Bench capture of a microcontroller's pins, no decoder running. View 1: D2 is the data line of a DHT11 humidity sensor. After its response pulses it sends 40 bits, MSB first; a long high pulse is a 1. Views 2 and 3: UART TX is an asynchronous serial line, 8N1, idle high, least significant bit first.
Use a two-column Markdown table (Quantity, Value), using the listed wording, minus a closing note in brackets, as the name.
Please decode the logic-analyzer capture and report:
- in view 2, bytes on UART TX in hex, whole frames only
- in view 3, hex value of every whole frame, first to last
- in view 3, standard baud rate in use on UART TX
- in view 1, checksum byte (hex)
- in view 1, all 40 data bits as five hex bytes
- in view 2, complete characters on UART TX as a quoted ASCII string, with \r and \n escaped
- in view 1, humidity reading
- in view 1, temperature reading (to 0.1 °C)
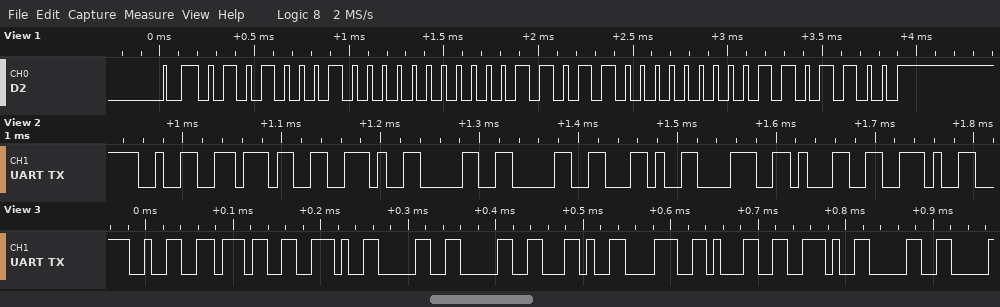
| Quantity | Value |
|---|---|
| in view 2, bytes on UART TX in hex, whole frames only | 32 37 2E 30 30 2C 38 31 2E |
| in view 3, hex value of every whole frame, first to last | 32 37 2E 30 30 2C 38 31 2E 30 |
| in view 3, standard baud rate in use on UART TX | 115200 baud |
| in view 1, checksum byte | 0x6C |
| in view 1, all 40 data bits as five hex bytes | 51 00 1B 00 6C |
| in view 2, complete characters on UART TX as a quoted ASCII string, with \r and \n escaped | "27.00,81." |
| in view 1, humidity reading | 81 % |
| in view 1, temperature reading | 27.0 °C |
